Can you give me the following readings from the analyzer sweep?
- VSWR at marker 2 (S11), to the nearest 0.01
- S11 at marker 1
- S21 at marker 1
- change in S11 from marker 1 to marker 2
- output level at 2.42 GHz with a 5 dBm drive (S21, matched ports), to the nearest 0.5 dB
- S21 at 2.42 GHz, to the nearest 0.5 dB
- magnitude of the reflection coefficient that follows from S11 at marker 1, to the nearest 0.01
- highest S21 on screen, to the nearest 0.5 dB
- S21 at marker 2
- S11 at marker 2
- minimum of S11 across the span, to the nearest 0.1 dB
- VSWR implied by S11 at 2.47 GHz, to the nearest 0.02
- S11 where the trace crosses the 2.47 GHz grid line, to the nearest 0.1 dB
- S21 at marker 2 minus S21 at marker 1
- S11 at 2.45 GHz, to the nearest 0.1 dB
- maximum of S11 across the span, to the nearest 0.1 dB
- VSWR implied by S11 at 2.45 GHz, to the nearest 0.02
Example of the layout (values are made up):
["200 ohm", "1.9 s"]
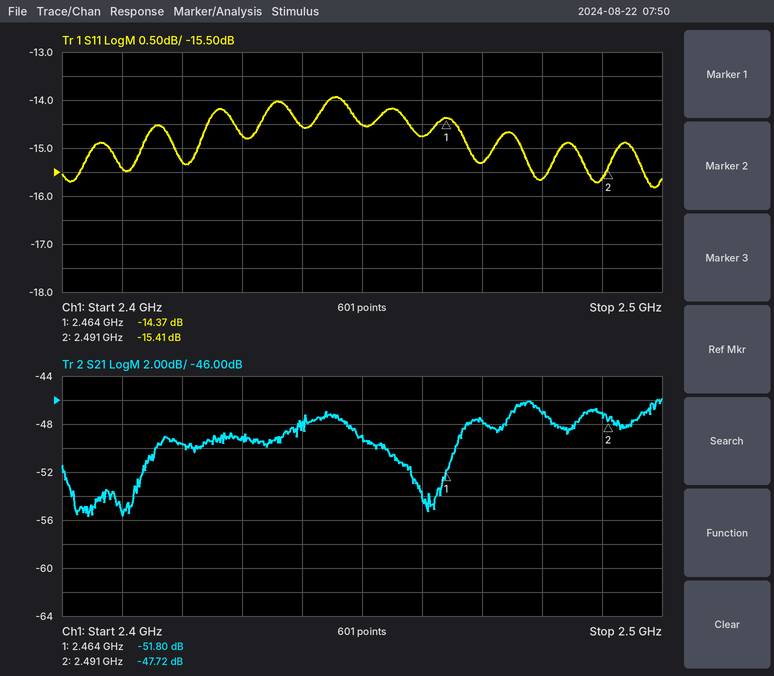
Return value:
["1.41", "-14.37 dB", "-51.80 dB", "-1.04 dB", "-44.5 dBm", "-49.5 dB", "0.19", "-46.0 dB", "-47.72 dB", "-15.41 dB", "-15.8 dB", "1.42", "-15.3 dB", "4.08 dB", "-14.5 dB", "-13.9 dB", "1.46"]
